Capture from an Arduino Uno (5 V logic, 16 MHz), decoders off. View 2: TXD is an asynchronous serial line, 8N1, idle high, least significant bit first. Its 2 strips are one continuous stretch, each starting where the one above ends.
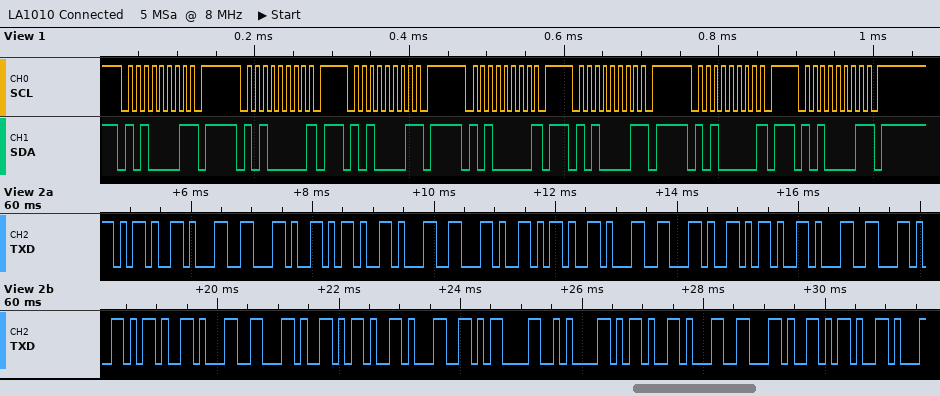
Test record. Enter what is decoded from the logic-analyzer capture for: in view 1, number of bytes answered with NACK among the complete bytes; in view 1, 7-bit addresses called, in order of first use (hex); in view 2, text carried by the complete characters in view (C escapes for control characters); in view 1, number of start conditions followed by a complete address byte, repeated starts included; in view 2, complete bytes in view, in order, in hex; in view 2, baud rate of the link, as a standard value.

7
0x50
"-1,-1,-1,-1,-1,-1\r\n-1,-"
7
2D 31 2C 2D 31 2C 2D 31 2C 2D 31 2C 2D 31 2C 2D 31 0D 0A 2D 31 2C 2D
9600 baud
